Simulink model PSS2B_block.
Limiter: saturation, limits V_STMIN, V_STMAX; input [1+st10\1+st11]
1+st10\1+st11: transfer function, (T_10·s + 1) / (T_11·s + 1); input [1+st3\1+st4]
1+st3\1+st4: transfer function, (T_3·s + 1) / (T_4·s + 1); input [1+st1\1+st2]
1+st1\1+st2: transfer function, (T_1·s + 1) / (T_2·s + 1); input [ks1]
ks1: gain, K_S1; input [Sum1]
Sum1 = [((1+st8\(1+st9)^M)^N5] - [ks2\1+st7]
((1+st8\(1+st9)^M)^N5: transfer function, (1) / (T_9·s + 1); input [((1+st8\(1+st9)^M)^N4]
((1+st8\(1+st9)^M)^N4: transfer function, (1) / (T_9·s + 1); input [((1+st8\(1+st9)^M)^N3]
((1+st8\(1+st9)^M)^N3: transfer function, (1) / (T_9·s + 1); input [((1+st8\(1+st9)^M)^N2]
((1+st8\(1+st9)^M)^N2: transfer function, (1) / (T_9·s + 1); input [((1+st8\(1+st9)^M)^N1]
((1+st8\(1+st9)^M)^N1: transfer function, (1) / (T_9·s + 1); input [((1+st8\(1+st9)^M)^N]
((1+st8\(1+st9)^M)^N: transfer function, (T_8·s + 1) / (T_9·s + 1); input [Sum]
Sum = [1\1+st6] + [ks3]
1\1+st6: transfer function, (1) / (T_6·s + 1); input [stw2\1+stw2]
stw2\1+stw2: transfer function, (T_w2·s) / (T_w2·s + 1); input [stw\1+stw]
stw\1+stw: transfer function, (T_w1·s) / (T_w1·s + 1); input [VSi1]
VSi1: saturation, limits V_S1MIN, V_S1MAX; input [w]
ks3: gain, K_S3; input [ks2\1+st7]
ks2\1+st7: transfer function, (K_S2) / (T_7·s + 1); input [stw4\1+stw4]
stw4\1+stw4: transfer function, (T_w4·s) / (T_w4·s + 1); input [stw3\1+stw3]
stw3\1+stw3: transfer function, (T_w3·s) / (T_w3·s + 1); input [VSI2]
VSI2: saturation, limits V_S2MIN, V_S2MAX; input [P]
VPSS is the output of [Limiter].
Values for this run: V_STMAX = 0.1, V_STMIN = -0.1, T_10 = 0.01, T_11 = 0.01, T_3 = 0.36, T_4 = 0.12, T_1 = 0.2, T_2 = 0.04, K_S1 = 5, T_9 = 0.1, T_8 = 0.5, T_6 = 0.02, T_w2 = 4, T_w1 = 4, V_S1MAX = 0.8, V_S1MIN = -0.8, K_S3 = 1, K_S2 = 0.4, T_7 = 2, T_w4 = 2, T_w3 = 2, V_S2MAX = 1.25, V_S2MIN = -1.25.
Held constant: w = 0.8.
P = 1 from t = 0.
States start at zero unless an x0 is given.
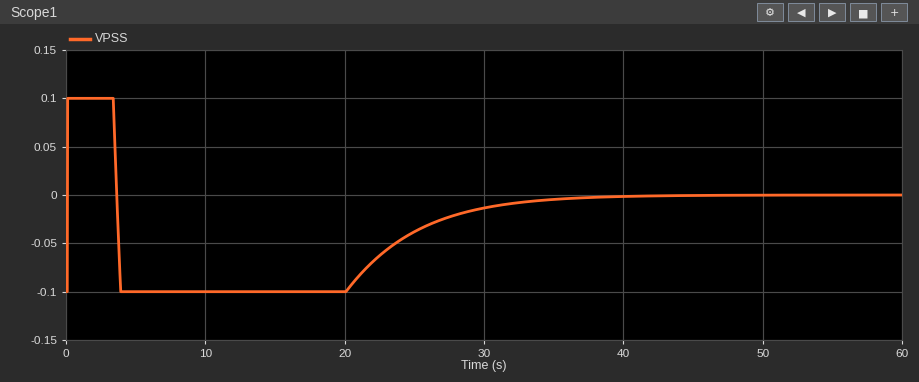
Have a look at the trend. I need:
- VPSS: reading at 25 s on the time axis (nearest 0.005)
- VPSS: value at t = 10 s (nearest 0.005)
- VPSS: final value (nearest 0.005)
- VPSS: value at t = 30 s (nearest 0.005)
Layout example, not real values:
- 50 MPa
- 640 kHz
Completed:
- -0.040
- -0.100
- 0.000
- -0.015
